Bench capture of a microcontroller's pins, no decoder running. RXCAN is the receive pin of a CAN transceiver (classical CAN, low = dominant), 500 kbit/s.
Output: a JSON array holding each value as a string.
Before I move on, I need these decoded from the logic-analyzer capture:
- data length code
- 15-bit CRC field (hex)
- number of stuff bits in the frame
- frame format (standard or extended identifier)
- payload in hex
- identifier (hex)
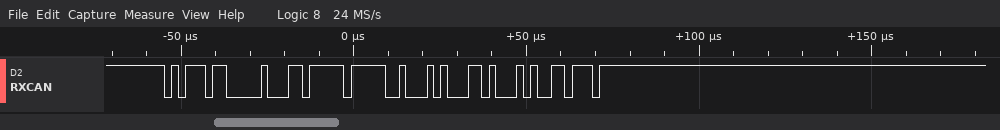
["3", "0x229B", "3", "standard", "7F E8 A3", "0x5D8"]
